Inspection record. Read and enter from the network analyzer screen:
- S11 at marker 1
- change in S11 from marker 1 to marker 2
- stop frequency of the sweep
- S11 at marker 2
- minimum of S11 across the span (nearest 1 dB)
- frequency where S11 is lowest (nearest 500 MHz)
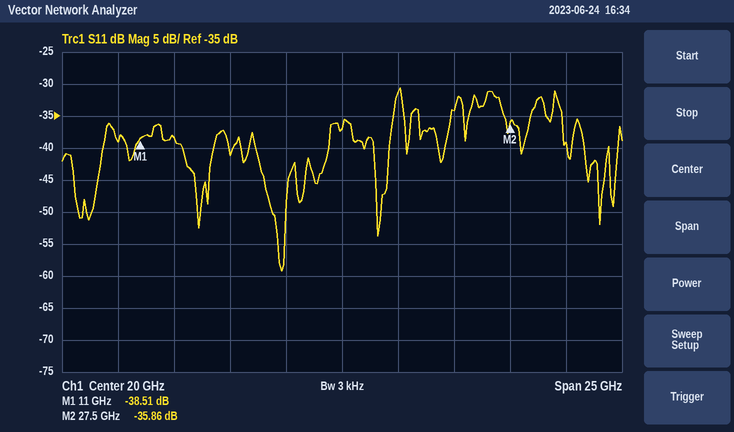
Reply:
-38.51 dB
2.65 dB
32.5 GHz
-35.86 dB
-59 dB
17.5 GHz
